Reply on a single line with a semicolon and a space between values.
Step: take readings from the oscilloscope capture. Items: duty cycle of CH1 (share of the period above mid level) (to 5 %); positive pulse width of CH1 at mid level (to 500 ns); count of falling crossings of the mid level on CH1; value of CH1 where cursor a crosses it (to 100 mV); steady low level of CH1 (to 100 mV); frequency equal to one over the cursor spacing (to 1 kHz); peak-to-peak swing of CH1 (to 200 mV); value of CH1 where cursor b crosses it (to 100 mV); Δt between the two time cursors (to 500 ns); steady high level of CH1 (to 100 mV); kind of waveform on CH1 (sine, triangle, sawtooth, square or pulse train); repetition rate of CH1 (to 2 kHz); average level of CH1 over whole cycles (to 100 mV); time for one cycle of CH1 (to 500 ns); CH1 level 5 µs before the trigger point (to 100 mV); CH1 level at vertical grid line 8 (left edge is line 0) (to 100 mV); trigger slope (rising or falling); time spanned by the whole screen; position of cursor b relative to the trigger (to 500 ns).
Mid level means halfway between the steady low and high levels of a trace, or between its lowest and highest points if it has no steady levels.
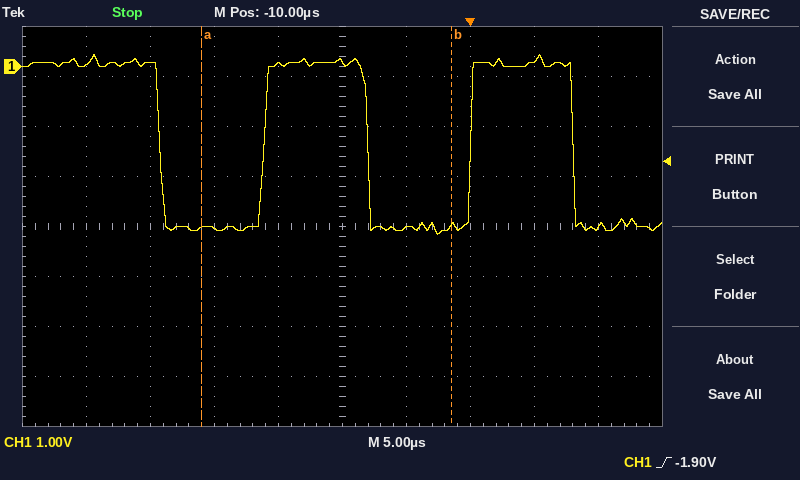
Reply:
50 %; 8.0 µs; 3; -3.2 V; -3.2 V; 51 kHz; 3.6 V; -3.2 V; 19.5 µs; 100 mV; square; 62 kHz; -1.6 V; 16.0 µs; -3.2 V; 100 mV; rising; 50 µs; -1.5 µs
